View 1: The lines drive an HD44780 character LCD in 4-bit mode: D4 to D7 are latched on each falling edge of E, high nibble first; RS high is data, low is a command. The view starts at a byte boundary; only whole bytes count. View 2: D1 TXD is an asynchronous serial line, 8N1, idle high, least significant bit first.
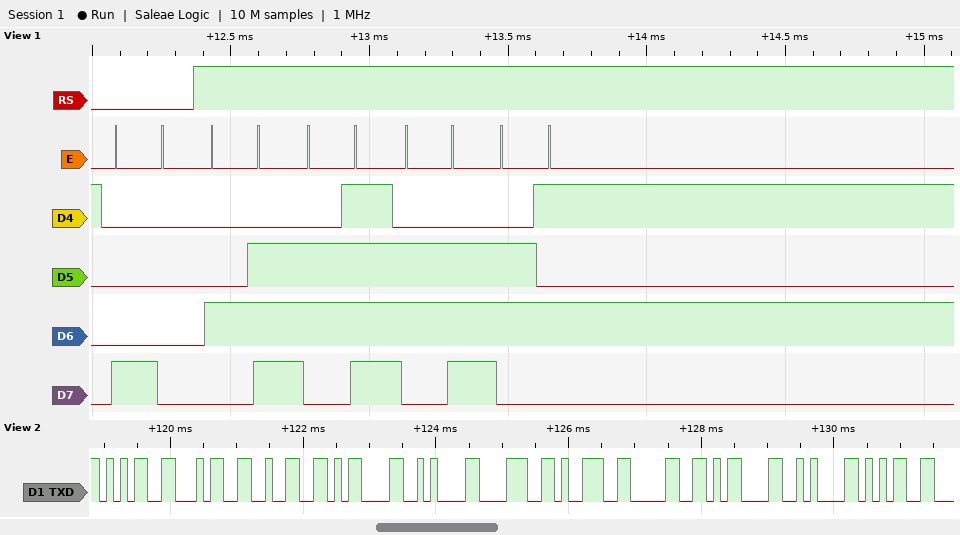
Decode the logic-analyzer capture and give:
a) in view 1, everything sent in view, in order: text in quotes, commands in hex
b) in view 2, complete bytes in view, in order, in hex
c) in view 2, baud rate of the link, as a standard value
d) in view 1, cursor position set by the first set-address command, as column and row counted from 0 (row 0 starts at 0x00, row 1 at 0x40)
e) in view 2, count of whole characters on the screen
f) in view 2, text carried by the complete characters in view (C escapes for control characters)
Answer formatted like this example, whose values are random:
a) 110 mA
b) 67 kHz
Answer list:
a) 0x80 "None"
b) 0x35 0x34 0x32 0x0D 0x0A 0x38 0x39 0x30 0x0D 0x0A 0x35
c) 9600 baud
d) column 0, row 0
e) 11
f) "542\r\n890\r\n5"
